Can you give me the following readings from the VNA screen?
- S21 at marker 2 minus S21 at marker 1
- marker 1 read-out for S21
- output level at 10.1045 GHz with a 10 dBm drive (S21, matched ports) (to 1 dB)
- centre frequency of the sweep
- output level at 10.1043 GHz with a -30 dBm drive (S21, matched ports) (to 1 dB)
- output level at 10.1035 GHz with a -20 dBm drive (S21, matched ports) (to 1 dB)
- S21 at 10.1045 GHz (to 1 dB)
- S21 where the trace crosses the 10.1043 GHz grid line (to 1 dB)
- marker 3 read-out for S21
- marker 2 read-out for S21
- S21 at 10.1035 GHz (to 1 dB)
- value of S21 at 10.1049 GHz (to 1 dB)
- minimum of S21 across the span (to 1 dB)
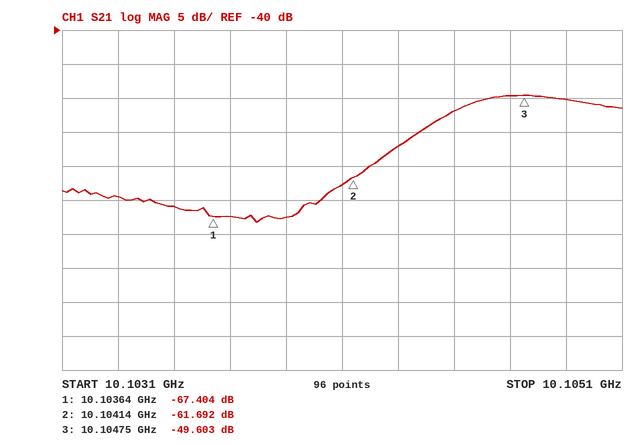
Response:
5.712 dB
-67.404 dB
-42 dBm
10.1041 GHz
-87 dBm
-86 dBm
-52 dB
-57 dB
-49.603 dB
-61.692 dB
-66 dB
-50 dB
-68 dB
